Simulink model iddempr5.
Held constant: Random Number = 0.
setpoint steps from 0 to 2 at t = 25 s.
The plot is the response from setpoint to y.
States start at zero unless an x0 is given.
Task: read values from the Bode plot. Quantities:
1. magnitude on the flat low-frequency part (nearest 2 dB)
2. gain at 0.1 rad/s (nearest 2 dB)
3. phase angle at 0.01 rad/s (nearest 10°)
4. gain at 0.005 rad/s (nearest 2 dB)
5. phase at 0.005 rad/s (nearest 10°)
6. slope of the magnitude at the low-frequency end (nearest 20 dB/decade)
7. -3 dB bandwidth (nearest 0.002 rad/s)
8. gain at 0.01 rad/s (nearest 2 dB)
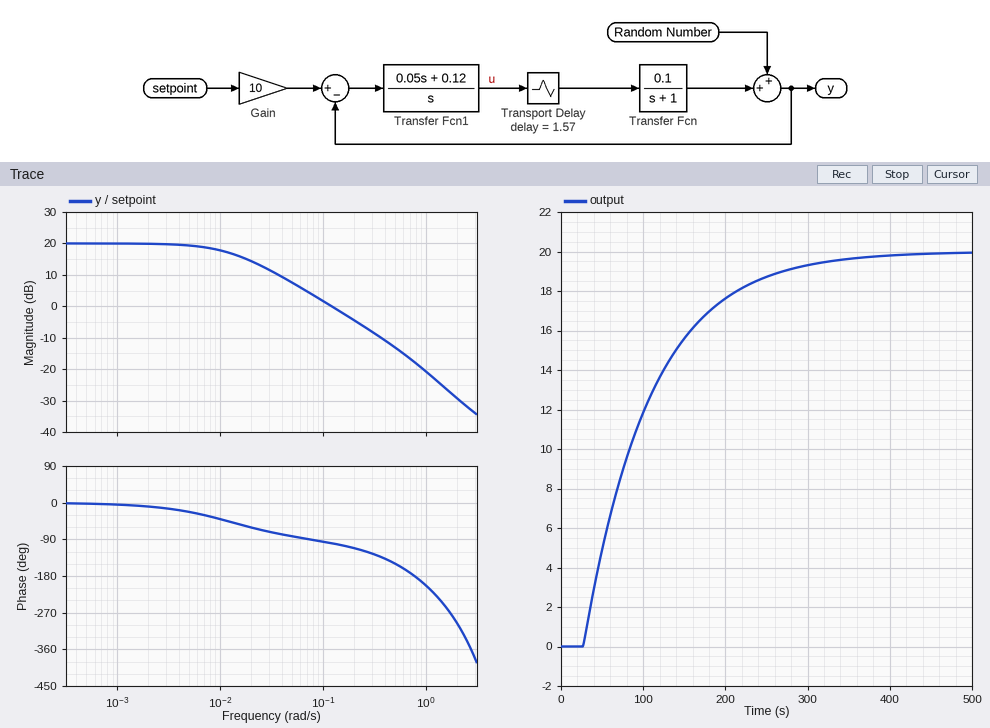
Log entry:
20 dB
2 dB
-40°
20 dB
-20°
0 dB/decade
0.012 rad/s
18 dB
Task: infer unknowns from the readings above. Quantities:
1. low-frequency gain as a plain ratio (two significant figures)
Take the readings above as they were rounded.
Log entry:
10
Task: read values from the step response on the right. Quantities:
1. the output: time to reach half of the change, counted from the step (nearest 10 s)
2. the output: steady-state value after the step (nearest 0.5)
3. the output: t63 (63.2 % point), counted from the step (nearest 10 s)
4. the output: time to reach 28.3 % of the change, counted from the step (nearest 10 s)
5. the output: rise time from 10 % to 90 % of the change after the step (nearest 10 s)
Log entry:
60 s
20.0
80 s
30 s
180 s
